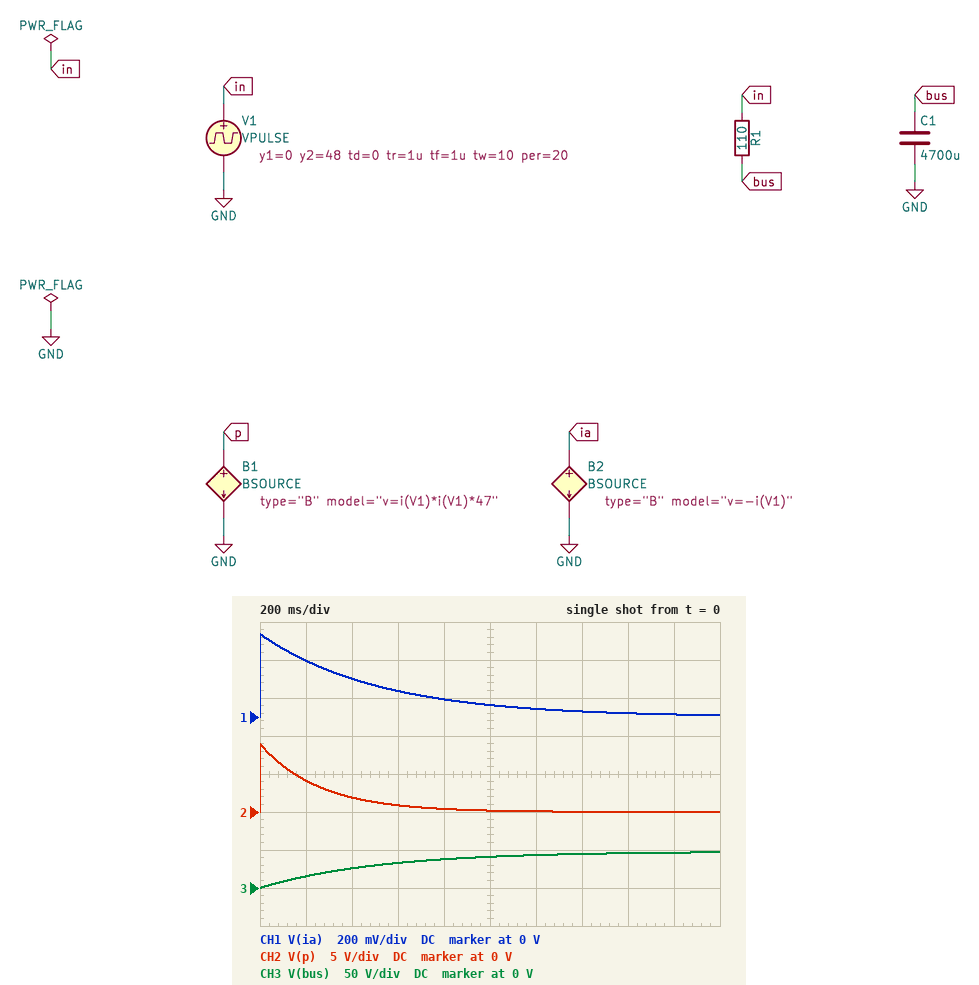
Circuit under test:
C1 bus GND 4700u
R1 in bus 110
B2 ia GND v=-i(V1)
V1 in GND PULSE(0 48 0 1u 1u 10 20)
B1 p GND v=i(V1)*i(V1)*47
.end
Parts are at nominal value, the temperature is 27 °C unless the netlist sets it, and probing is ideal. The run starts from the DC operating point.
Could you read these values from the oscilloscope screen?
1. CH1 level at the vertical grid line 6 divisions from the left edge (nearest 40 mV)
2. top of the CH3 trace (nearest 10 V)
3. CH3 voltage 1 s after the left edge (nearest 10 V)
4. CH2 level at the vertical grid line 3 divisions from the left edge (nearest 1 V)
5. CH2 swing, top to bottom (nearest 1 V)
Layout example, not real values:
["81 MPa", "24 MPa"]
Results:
["40 mV", "50 V", "40 V", "1 V", "9 V"]
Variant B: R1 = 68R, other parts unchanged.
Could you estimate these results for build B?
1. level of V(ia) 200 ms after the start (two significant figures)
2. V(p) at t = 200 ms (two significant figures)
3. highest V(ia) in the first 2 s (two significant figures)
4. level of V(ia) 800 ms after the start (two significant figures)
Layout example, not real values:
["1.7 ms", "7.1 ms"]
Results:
["380 mV", "6.7 V", "710 mV", "58 mV"]
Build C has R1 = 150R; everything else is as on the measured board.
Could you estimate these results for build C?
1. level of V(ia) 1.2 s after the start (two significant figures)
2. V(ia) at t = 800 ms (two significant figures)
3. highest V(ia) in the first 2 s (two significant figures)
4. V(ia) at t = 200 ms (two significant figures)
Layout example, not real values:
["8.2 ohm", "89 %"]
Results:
["58 mV", "100 mV", "320 mV", "240 mV"]
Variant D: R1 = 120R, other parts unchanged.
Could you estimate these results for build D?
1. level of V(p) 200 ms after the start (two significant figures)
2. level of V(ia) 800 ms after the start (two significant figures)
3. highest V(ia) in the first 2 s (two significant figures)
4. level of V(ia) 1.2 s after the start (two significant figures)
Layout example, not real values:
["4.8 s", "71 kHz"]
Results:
["3.7 V", "97 mV", "400 mV", "48 mV"]
